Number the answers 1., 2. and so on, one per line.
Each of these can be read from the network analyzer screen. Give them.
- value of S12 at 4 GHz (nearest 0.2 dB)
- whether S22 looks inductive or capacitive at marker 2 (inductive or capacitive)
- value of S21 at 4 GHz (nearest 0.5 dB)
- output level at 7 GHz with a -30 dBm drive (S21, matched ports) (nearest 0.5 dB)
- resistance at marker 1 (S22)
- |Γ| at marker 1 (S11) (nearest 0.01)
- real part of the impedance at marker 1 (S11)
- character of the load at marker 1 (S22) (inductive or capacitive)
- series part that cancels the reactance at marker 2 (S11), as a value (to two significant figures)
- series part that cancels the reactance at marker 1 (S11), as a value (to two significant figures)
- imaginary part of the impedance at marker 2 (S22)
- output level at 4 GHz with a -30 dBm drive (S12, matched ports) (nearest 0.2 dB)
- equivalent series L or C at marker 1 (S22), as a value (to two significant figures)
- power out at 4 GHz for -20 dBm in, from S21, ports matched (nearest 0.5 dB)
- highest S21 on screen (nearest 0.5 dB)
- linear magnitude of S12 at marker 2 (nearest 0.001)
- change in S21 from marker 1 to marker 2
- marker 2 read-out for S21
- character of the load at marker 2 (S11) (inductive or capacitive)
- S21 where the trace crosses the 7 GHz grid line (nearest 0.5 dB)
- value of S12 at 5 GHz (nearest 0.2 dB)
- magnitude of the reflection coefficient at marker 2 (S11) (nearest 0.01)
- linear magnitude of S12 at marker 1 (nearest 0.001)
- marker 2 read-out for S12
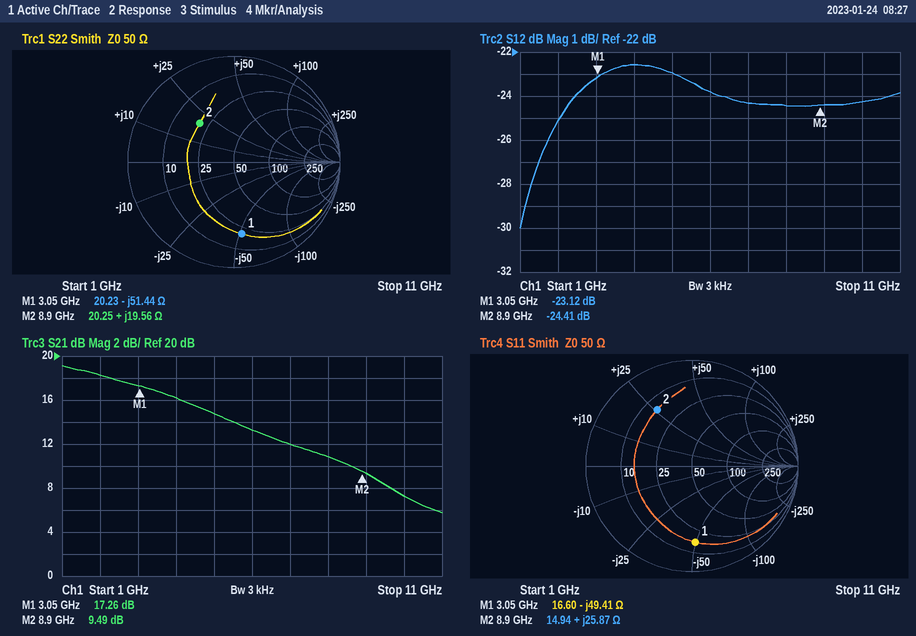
1. -22.6 dB
2. inductive
3. 16.0 dB
4. -18.0 dBm
5. 20.23 Ω
6. 0.72
7. 16.60 Ω
8. capacitive
9. 690 fF
10. 2.6 nH
11. +19.56 Ω
12. -52.6 dBm
13. 1.0 pF
14. -4.0 dBm
15. 19.0 dB
16. 0.060
17. -7.77 dB
18. 9.49 dB
19. inductive
20. 12.0 dB
21. -23.0 dB
22. 0.62
23. 0.070
24. -24.41 dB
